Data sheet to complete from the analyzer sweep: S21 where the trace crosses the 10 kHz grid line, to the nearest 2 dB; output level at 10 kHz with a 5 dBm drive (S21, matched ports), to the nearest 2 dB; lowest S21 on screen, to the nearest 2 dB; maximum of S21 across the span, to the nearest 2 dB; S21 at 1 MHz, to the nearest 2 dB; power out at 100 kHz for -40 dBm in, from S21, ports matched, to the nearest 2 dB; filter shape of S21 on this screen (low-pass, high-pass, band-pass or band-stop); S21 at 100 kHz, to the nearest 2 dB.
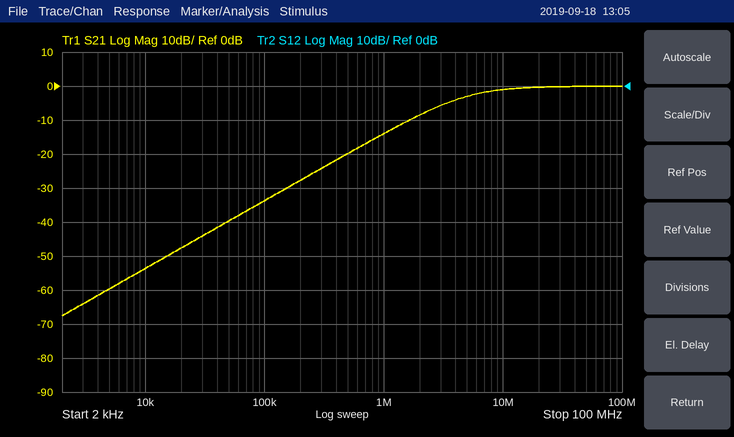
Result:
-54 dB
-48 dBm
-68 dB
0 dB
-14 dB
-74 dBm
high-pass
-34 dB
